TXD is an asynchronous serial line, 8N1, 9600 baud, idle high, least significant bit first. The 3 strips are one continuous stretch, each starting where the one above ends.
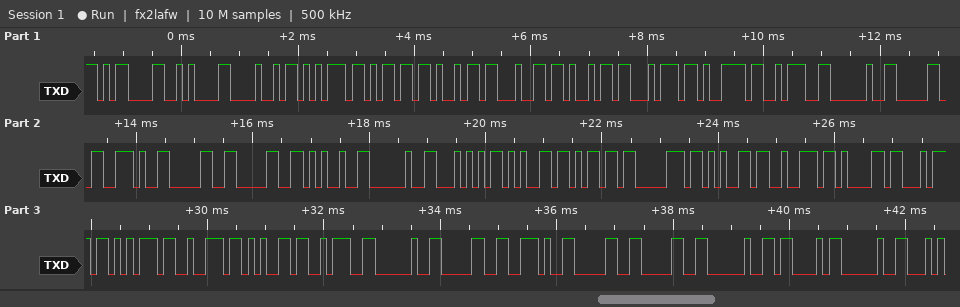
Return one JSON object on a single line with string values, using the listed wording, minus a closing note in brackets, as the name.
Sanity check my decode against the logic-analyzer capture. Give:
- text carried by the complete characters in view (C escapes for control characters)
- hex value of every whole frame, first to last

{"text carried by the complete characters in view": "\"\\r\\nHumidity: 0.00% Temperature: 0.00 C \"", "hex value of every whole frame, first to last": "0D 0A 48 75 6D 69 64 69 74 79 3A 20 30 2E 30 30 25 20 54 65 6D 70 65 72 61 74 75 72 65 3A 20 30 2E 30 30 20 43 20"}
